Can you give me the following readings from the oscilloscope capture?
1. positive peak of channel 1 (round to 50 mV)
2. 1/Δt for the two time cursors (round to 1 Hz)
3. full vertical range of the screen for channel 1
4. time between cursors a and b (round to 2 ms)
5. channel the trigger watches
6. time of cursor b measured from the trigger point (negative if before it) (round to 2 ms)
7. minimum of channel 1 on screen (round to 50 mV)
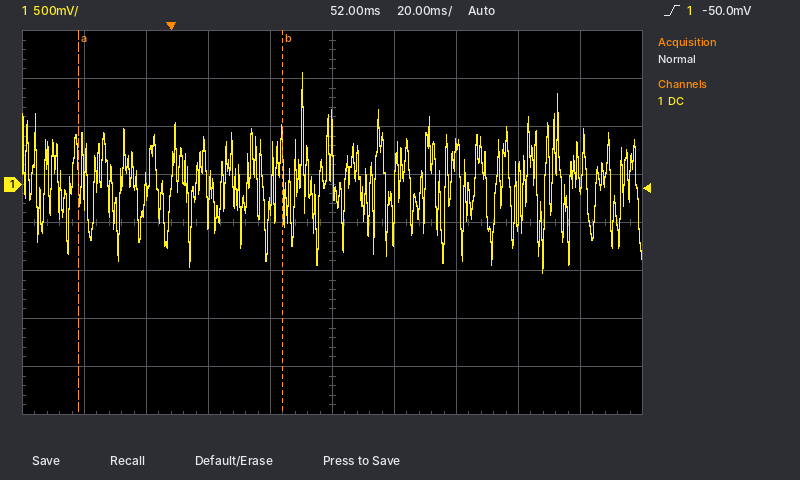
1.15 V
15 Hz
4 V
66 ms
channel 1
+36 ms
-900 mV
